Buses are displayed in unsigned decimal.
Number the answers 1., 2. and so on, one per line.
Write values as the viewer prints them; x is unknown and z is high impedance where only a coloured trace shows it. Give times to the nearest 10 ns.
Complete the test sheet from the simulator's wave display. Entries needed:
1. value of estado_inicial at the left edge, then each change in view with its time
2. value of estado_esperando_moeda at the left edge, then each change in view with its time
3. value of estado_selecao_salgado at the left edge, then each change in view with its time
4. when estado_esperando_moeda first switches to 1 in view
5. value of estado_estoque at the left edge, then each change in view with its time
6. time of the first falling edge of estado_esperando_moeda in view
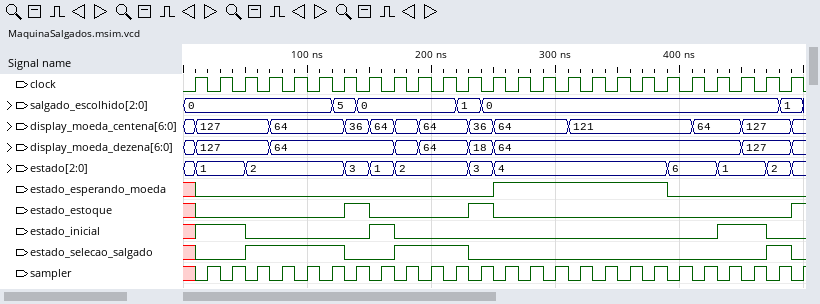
1. x, 1 at 10 ns, 0 at 50 ns, 1 at 150 ns, 0 at 170 ns, 1 at 430 ns, 0 at 470 ns
2. x, 0 at 10 ns, 1 at 250 ns, 0 at 390 ns
3. x, 0 at 10 ns, 1 at 50 ns, 0 at 130 ns, 1 at 170 ns, 0 at 230 ns, 1 at 470 ns, 0 at 490 ns
4. 250 ns
5. x, 0 at 10 ns, 1 at 130 ns, 0 at 150 ns, 1 at 230 ns, 0 at 250 ns, 1 at 490 ns
6. 390 ns
